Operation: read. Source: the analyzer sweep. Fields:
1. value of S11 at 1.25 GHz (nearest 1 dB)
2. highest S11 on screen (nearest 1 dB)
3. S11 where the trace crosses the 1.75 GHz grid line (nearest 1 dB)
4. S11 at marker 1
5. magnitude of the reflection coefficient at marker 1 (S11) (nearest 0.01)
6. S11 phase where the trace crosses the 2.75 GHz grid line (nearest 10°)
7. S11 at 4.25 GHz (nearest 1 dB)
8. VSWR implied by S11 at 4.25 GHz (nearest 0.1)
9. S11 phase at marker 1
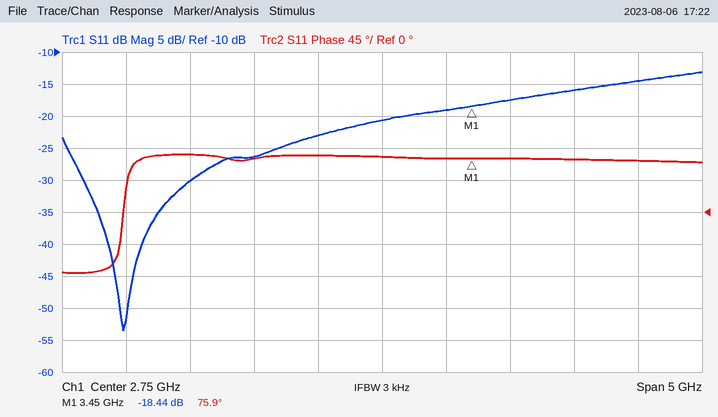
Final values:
-30 dB
-13 dB
-26 dB
-18.44 dB
0.12
80°
-16 dB
1.4
75.9°
